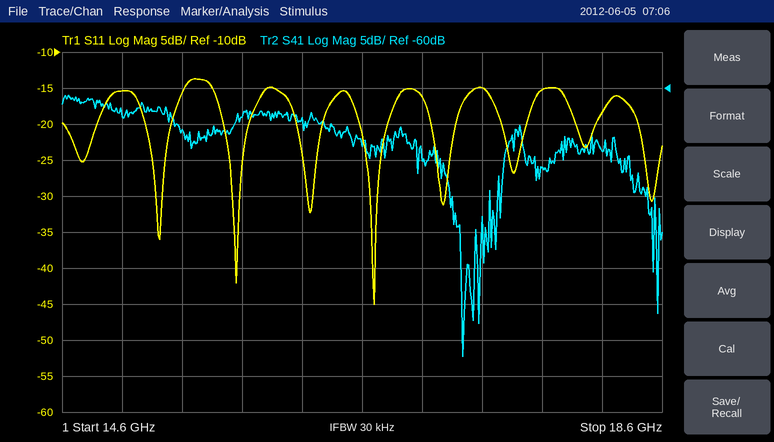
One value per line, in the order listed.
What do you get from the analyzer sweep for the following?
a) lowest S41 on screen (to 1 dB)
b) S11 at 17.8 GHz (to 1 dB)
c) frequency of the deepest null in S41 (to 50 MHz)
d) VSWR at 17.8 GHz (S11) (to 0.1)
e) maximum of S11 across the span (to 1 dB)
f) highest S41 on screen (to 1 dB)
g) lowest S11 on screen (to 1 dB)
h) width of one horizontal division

-97 dB
-15 dB
17.25 GHz
1.4
-14 dB
-61 dB
-45 dB
400 MHz
